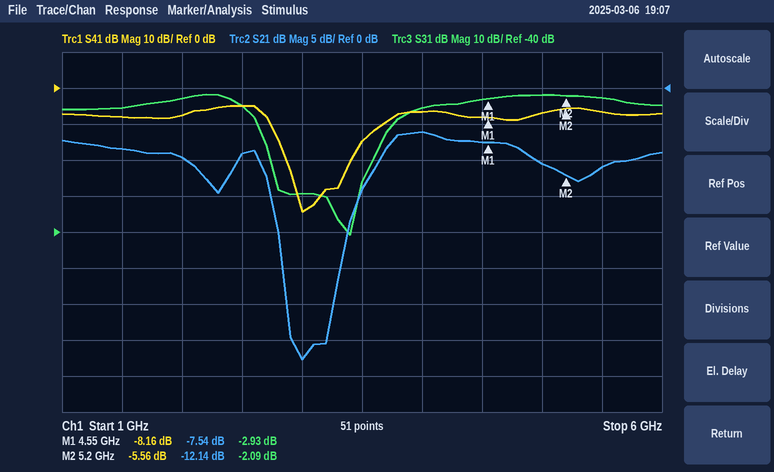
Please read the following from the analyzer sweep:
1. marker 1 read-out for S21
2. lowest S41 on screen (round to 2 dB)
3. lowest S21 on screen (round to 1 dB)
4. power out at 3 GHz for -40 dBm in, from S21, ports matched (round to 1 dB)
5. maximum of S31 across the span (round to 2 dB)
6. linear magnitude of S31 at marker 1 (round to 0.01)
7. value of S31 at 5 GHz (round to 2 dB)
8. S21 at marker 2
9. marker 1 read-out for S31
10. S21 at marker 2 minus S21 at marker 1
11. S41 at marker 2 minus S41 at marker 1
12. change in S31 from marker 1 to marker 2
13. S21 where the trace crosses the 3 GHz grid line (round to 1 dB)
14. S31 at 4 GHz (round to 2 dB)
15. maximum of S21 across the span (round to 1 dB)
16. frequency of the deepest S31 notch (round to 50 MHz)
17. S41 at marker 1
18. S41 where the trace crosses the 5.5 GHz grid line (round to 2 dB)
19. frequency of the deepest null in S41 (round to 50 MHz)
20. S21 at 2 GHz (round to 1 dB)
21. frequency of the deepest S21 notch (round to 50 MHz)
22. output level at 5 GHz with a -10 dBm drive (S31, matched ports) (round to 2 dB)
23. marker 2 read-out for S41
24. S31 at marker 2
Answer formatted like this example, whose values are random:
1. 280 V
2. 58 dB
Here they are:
1. -7.54 dB
2. -34 dB
3. -38 dB
4. -78 dBm
5. -2 dB
6. 0.71
7. -2 dB
8. -12.14 dB
9. -2.93 dB
10. -4.60 dB
11. 2.60 dB
12. 0.84 dB
13. -38 dB
14. -6 dB
15. -6 dB
16. 3.40 GHz
17. -8.16 dB
18. -6 dB
19. 3.00 GHz
20. -10 dB
21. 3.00 GHz
22. -12 dBm
23. -5.56 dB
24. -2.09 dB
